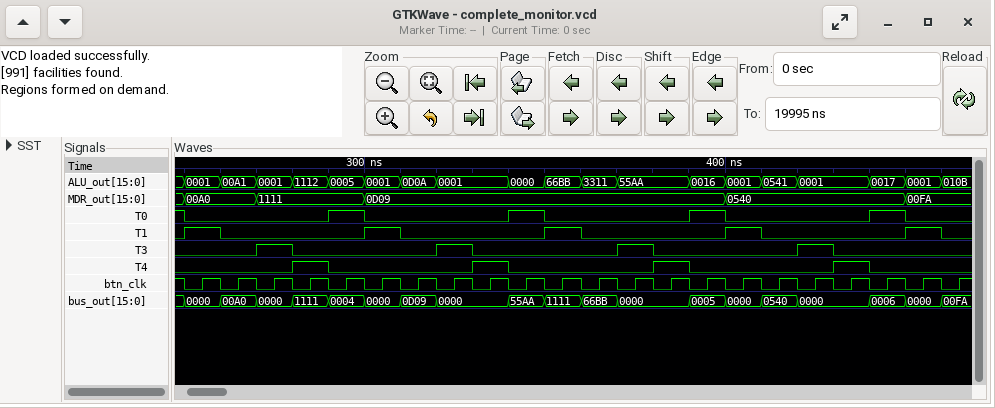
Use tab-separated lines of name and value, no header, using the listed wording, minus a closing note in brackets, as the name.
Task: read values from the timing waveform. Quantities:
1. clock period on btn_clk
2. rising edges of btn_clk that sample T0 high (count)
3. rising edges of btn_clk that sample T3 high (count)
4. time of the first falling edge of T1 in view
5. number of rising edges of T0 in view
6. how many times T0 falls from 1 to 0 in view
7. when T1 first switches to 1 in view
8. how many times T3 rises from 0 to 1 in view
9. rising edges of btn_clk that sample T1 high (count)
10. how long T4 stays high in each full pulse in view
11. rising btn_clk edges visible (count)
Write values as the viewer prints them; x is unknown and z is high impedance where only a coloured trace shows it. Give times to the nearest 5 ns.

clock period on btn_clk	10 ns
rising edges of btn_clk that sample T0 high	4
rising edges of btn_clk that sample T3 high	4
time of the first falling edge of T1 in view	260 ns
number of rising edges of T0 in view	4
how many times T0 falls from 1 to 0 in view	5
when T1 first switches to 1 in view	250 ns
how many times T3 rises from 0 to 1 in view	4
rising edges of btn_clk that sample T1 high	5
how long T4 stays high in each full pulse in view	10 ns, 10 ns, 10 ns, 10 ns
rising btn_clk edges visible	22
